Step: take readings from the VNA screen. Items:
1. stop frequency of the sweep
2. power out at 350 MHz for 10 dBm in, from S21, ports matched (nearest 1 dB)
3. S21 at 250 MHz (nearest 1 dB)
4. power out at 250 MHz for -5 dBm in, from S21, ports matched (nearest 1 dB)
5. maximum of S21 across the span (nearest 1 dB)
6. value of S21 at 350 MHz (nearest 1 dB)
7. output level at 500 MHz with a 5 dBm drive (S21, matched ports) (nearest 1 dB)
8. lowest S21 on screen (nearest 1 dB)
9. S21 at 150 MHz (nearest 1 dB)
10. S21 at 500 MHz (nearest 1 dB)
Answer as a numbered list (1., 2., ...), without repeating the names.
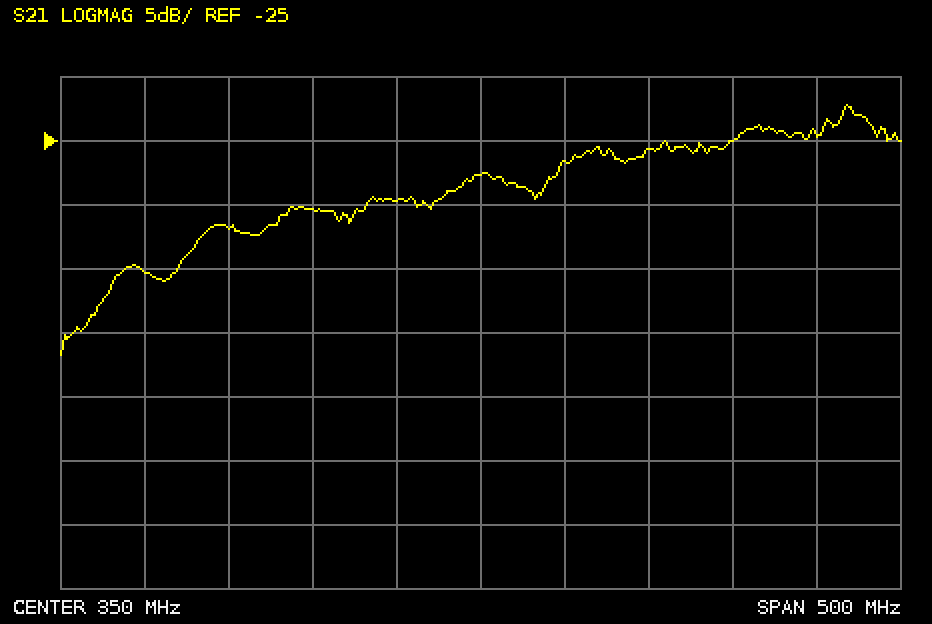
1. 600 MHz
2. -18 dBm
3. -30 dB
4. -35 dBm
5. -22 dB
6. -28 dB
7. -20 dBm
8. -42 dB
9. -35 dB
10. -25 dB
